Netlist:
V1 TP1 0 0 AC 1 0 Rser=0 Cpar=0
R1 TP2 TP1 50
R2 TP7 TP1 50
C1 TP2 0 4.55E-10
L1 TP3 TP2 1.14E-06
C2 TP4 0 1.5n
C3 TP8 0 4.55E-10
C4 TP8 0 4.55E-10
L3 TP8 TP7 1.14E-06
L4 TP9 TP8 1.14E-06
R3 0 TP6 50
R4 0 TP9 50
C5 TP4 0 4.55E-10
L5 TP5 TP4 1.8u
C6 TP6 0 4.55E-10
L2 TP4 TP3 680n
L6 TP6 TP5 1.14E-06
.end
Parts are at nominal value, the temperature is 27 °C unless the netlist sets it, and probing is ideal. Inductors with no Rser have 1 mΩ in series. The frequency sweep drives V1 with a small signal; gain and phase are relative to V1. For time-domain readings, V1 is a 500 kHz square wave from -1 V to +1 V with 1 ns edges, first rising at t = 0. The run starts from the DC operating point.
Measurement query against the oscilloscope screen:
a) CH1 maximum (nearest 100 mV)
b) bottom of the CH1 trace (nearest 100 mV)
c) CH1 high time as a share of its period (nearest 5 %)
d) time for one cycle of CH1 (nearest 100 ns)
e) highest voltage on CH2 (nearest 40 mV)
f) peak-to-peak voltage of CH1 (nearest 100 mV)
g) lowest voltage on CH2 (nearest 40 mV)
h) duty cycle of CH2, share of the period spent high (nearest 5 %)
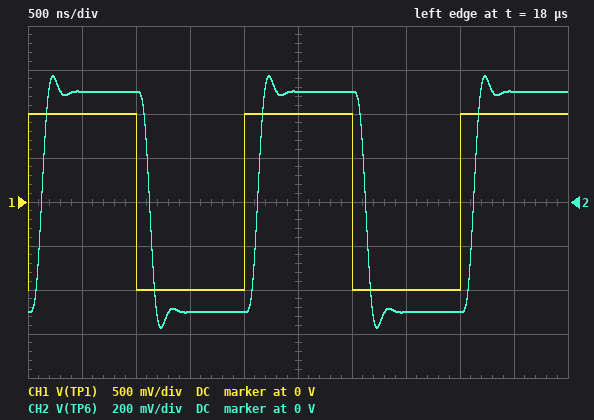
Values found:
1.0 V
-1.0 V
50 %
2.0 µs
560 mV
2.0 V
-560 mV
50 %
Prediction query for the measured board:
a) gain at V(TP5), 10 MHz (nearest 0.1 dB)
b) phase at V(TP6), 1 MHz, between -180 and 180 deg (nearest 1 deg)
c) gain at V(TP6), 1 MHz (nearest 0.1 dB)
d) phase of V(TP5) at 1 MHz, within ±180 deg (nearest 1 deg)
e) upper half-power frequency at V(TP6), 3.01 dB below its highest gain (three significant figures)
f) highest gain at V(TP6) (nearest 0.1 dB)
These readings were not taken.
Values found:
-34.7 dB
-43 deg
-6.1 dB
-35 deg
3.98 MHz
-6.0 dB
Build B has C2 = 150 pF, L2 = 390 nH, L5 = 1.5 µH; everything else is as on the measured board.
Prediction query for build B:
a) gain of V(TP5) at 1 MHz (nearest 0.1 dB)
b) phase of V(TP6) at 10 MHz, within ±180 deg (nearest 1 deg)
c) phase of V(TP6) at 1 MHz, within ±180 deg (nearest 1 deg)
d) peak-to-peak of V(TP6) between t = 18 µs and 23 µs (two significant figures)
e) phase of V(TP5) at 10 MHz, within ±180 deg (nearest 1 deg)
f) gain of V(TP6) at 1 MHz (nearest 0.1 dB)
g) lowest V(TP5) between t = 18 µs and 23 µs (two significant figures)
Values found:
-6.1 dB
11 deg
-29 deg
1.2 V
137 deg
-6.0 dB
-550 mV
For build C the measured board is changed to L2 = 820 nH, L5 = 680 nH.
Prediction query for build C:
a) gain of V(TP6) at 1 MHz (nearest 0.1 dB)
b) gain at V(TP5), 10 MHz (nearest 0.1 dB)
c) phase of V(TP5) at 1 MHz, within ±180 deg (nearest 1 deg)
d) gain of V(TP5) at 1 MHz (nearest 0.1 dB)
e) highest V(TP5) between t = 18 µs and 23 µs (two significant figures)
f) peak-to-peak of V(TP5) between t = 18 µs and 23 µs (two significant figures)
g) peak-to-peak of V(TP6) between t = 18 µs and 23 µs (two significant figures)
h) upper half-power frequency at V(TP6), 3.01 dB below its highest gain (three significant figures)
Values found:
-6.2 dB
-30.3 dB
-31 deg
-6.3 dB
520 mV
1.0 V
1.1 V
4.80 MHz
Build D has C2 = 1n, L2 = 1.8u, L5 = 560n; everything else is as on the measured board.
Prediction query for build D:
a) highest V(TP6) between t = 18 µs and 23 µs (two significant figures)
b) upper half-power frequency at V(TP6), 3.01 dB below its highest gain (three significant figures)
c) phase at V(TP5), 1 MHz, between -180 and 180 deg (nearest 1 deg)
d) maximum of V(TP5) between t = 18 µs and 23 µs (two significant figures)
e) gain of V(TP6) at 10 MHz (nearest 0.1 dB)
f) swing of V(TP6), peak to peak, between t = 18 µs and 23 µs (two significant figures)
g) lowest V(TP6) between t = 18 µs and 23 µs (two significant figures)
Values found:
600 mV
4.82 MHz
-30 deg
550 mV
-35.8 dB
1.2 V
-600 mV
